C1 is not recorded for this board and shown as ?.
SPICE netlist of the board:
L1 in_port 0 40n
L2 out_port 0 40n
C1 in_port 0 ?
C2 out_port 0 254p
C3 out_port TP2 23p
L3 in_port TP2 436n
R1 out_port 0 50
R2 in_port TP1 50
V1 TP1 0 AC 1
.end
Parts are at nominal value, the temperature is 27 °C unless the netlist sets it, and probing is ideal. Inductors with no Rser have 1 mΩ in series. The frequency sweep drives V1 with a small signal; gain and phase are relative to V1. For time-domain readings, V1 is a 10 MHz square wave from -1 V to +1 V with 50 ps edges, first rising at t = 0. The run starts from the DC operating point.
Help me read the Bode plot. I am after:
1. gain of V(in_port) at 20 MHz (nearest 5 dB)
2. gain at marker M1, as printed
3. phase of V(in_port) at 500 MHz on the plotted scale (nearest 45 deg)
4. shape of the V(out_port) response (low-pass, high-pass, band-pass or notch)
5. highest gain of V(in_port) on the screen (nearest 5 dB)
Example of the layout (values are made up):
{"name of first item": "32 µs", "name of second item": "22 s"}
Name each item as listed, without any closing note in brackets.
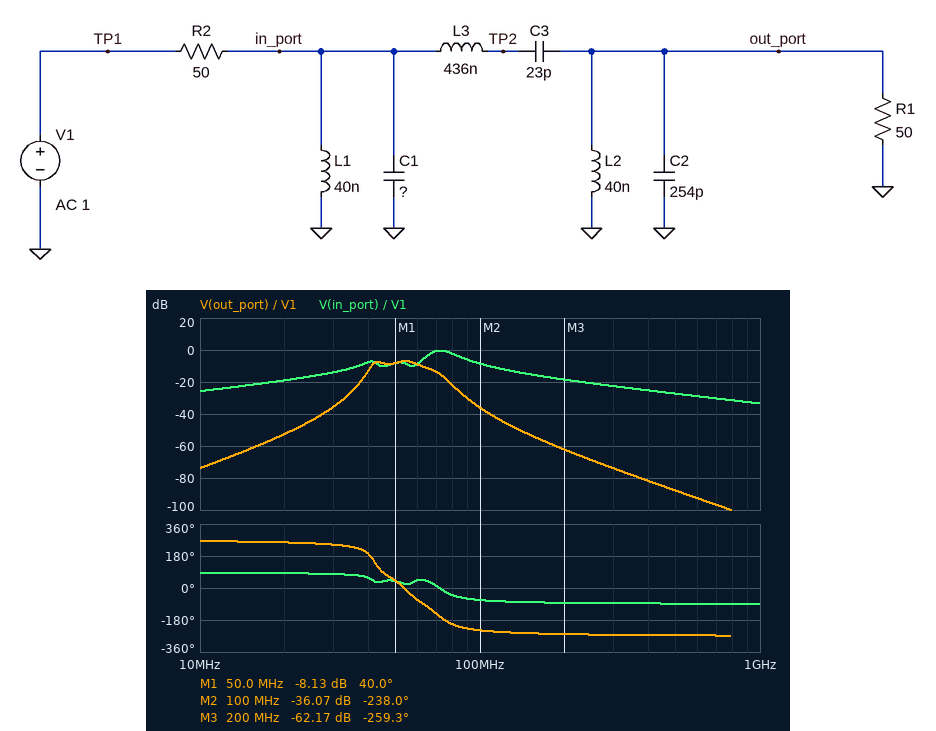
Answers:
{"gain of V(in_port) at 20 MHz": "-20 dB", "gain at marker M1, as printed": "-8.13 dB", "phase of V(in_port) at 500 MHz on the plotted scale": "-90 deg", "shape of the V(out_port) response": "band-pass", "highest gain of V(in_port) on the screen": "0 dB"}
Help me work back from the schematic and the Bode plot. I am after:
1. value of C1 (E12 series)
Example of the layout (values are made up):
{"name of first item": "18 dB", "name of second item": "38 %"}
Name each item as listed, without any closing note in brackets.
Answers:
{"value of C1": "150 pF"}
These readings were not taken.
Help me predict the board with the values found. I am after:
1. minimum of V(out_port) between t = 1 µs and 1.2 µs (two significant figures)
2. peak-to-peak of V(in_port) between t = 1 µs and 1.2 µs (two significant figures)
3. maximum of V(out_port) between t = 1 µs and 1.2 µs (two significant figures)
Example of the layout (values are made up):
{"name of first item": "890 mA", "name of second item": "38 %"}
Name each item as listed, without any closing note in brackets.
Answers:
{"minimum of V(out_port) between t = 1 µs and 1.2 µs": "-140 mV", "peak-to-peak of V(in_port) between t = 1 µs and 1.2 µs": "1.1 V", "maximum of V(out_port) between t = 1 µs and 1.2 µs": "140 mV"}
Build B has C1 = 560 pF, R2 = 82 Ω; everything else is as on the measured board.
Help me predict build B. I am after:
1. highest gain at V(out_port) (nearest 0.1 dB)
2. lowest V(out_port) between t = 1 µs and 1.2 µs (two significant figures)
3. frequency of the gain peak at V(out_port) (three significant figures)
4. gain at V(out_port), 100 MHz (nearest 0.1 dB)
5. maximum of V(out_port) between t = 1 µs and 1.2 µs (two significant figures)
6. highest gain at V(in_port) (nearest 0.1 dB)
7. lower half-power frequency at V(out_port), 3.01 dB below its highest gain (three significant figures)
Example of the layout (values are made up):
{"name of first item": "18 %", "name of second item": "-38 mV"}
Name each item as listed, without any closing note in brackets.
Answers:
{"highest gain at V(out_port)": "-15.1 dB", "lowest V(out_port) between t = 1 µs and 1.2 µs": "-48 mV", "frequency of the gain peak at V(out_port)": "44.9 MHz", "gain at V(out_port), 100 MHz": "-55.6 dB", "maximum of V(out_port) between t = 1 µs and 1.2 µs": "48 mV", "highest gain at V(in_port)": "-0.2 dB", "lower half-power frequency at V(out_port), 3.01 dB below its highest gain": "41.4 MHz"}
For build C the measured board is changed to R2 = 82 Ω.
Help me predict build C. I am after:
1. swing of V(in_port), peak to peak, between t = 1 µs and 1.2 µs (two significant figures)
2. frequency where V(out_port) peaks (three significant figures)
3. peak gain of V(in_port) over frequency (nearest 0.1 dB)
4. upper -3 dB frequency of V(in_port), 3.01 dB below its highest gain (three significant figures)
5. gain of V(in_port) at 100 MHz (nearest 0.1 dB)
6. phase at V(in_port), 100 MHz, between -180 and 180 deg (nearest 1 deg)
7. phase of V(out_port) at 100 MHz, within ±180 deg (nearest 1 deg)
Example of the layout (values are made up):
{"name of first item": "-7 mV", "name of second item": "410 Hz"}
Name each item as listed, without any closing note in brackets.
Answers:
{"swing of V(in_port), peak to peak, between t = 1 µs and 1.2 µs": "770 mV", "frequency where V(out_port) peaks": "54.0 MHz", "peak gain of V(in_port) over frequency": "-0.5 dB", "upper -3 dB frequency of V(in_port), 3.01 dB below its highest gain": "77.9 MHz", "gain of V(in_port) at 100 MHz": "-12.4 dB", "phase at V(in_port), 100 MHz, between -180 and 180 deg": "-76 deg", "phase of V(out_port) at 100 MHz, within ±180 deg": "114 deg"}
